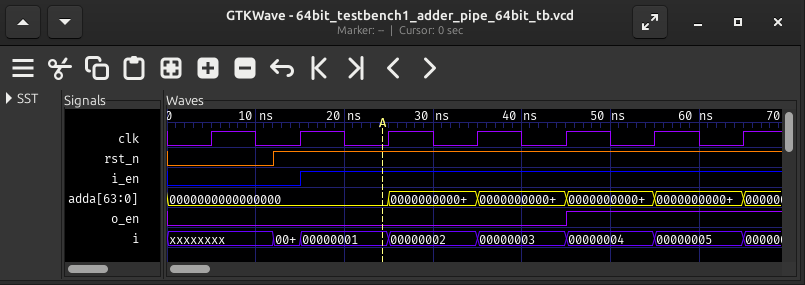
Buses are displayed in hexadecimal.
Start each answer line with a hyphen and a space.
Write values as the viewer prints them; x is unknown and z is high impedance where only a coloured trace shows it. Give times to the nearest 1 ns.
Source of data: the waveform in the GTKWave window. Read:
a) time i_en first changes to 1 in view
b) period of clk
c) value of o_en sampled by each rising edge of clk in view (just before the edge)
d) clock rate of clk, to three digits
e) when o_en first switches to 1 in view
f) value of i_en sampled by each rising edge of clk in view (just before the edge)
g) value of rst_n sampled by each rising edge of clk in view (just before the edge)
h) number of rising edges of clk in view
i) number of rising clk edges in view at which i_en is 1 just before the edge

- 15 ns
- 10 ns
- 0 0 0 0 0 1 1
- 100 MHz
- 45 ns
- 0 0 1 1 1 1 1
- 0 1 1 1 1 1 1
- 7
- 5
